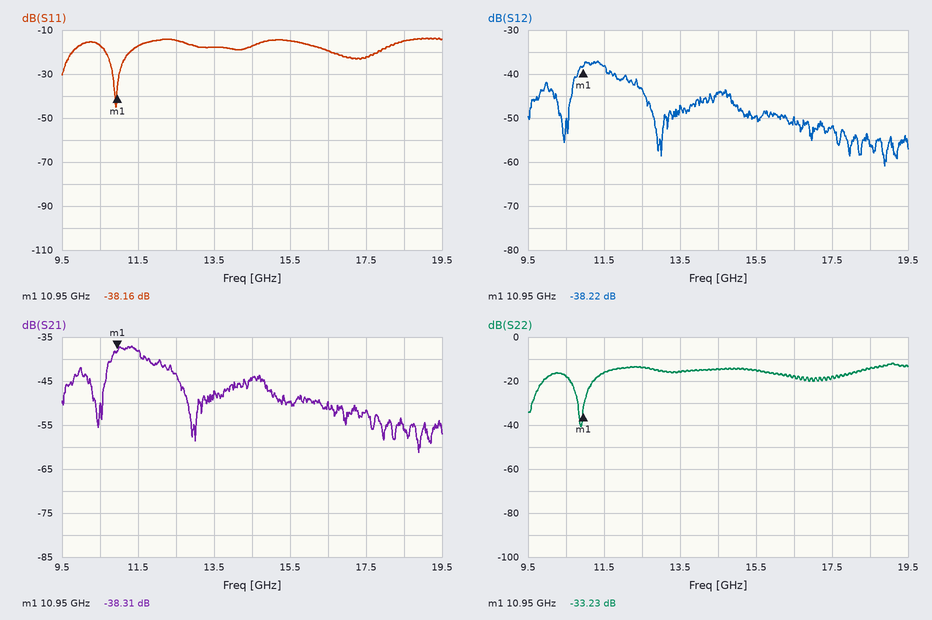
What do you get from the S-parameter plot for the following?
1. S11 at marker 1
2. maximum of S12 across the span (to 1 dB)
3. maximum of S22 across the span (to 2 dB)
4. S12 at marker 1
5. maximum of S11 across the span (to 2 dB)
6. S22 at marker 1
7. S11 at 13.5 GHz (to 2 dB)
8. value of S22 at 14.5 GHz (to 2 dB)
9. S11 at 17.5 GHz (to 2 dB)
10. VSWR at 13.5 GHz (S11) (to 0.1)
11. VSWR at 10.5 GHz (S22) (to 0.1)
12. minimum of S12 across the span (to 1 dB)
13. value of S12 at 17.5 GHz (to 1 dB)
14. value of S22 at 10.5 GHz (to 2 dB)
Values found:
-38.16 dB
-37 dB
-12 dB
-38.22 dB
-14 dB
-33.23 dB
-18 dB
-14 dB
-22 dB
1.3
1.3
-61 dB
-52 dB
-18 dB
